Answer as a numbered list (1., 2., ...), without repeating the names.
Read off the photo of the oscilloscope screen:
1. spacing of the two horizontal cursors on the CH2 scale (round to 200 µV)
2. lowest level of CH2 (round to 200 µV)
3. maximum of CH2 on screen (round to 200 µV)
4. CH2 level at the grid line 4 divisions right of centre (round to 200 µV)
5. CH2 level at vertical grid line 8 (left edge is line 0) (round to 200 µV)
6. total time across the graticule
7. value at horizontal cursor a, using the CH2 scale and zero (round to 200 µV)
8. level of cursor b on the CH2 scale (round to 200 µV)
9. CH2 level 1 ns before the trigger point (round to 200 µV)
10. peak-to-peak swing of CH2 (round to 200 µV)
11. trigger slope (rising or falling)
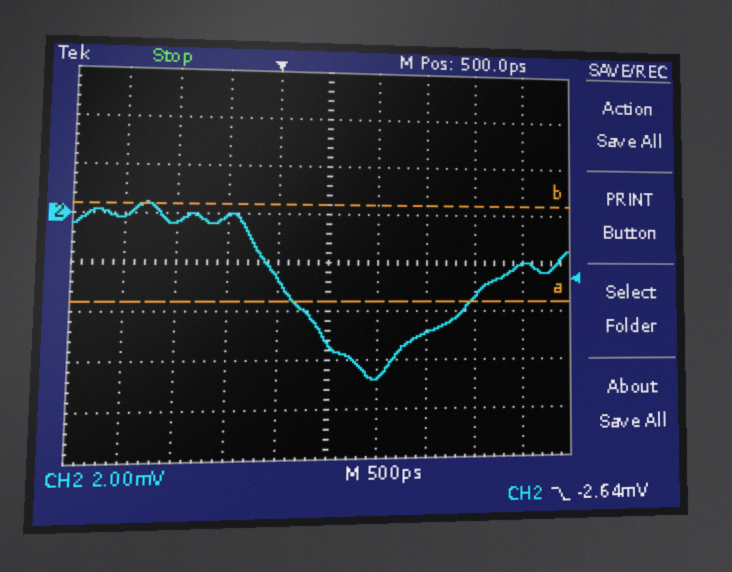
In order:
1. 4.0 mV
2. -6.8 mV
3. 400 µV
4. -2.0 mV
5. -3.4 mV
6. 5 ns
7. -3.6 mV
8. 400 µV
9. -400 µV
10. 7.2 mV
11. falling
